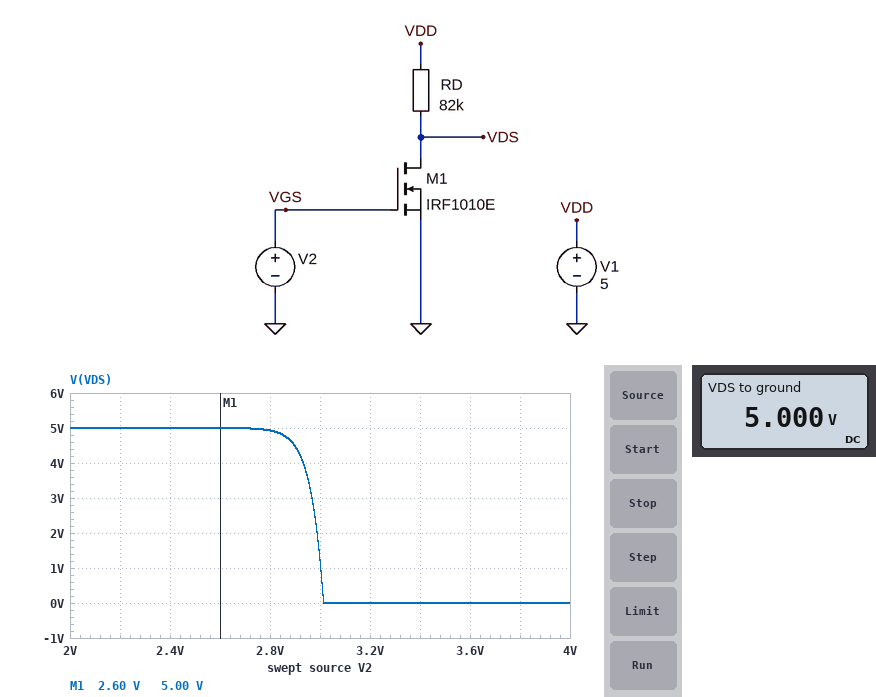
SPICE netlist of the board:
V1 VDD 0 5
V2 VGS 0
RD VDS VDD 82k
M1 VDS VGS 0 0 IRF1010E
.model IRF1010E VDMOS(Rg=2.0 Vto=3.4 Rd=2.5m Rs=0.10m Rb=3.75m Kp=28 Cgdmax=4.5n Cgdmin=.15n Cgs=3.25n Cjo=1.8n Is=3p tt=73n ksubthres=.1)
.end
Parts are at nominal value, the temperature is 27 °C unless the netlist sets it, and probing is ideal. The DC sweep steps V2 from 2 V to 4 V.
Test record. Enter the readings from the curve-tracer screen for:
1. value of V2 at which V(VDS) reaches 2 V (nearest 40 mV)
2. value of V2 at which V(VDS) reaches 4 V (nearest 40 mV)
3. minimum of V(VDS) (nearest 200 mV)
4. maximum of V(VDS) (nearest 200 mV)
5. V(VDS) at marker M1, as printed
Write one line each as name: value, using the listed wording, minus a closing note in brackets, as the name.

value of V2 at which V(VDS) reaches 2 V: 3.00 V
value of V2 at which V(VDS) reaches 4 V: 2.92 V
minimum of V(VDS): 0 V
maximum of V(VDS): 5.0 V
V(VDS) at marker M1, as printed: 5.00 V
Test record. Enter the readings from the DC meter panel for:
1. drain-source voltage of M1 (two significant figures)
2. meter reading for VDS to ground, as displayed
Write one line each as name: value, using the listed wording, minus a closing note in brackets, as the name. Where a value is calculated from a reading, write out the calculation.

drain-source voltage of M1: 5 V = 5.0 V
meter reading for VDS to ground, as displayed: 5.000 V
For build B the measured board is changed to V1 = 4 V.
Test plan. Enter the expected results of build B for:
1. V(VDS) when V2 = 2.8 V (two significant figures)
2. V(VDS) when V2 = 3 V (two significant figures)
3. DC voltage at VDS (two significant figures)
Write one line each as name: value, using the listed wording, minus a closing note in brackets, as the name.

V(VDS) when V2 = 2.8 V: 3.9 V
V(VDS) when V2 = 3 V: 220 mV
DC voltage at VDS: 4.0 V
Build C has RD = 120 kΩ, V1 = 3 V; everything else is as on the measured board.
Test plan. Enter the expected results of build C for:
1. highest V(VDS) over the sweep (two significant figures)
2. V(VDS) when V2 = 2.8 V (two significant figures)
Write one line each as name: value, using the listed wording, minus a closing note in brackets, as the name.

highest V(VDS) over the sweep: 3.0 V
V(VDS) when V2 = 2.8 V: 2.9 V
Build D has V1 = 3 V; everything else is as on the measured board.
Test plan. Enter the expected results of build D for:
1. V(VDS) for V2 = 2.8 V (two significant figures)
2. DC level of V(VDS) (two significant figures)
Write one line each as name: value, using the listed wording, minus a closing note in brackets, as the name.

V(VDS) for V2 = 2.8 V: 2.9 V
DC level of V(VDS): 3.0 V
